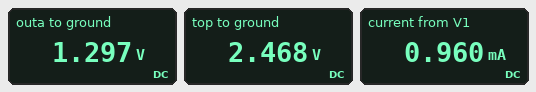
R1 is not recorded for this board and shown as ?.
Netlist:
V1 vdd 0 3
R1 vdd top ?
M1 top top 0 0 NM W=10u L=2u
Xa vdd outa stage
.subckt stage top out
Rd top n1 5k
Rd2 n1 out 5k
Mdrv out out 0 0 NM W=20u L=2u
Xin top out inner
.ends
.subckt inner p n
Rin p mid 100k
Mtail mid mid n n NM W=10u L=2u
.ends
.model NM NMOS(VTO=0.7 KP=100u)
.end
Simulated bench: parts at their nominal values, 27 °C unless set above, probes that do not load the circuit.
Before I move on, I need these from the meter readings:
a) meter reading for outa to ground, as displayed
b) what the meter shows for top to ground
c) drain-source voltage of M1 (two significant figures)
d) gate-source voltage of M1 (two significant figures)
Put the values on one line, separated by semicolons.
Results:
1.297 V; 2.468 V; 2.5 V; 2.5 V
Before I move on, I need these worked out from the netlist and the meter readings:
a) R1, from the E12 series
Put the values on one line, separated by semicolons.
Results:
680 Ω
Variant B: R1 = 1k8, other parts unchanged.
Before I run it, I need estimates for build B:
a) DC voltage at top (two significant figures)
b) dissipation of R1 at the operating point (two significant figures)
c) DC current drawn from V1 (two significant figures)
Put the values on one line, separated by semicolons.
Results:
2.1 V; 440 µW; 670 µA
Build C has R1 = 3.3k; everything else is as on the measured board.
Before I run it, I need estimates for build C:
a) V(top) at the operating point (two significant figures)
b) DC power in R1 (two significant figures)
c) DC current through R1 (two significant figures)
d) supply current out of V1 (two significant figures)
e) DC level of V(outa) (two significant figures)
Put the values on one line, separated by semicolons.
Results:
1.9 V; 390 µW; 340 µA; 520 µA; 1.3 V
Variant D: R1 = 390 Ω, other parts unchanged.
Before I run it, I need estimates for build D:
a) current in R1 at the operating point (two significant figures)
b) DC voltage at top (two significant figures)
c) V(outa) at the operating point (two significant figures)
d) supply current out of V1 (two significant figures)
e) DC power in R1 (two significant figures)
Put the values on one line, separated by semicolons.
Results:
940 µA; 2.6 V; 1.3 V; 1.1 mA; 340 µW
